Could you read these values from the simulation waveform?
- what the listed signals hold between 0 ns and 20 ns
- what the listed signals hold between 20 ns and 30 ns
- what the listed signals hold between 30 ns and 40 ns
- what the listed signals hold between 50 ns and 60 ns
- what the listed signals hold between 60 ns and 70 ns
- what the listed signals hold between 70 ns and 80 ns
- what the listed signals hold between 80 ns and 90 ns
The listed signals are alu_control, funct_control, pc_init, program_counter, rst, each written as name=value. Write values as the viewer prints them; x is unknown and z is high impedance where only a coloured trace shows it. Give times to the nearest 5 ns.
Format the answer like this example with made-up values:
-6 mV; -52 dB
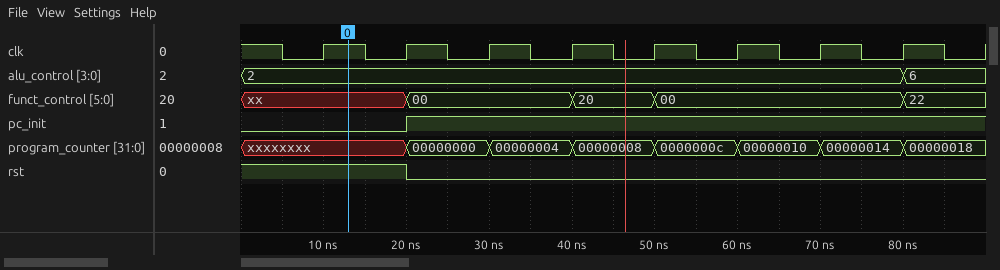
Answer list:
alu_control=2, funct_control=xx, pc_init=0, program_counter=xxxxxxxx, rst=1; alu_control=2, funct_control=00, pc_init=1, program_counter=00000000, rst=0; alu_control=2, funct_control=00, pc_init=1, program_counter=00000004, rst=0; alu_control=2, funct_control=00, pc_init=1, program_counter=0000000c, rst=0; alu_control=2, funct_control=00, pc_init=1, program_counter=00000010, rst=0; alu_control=2, funct_control=00, pc_init=1, program_counter=00000014, rst=0; alu_control=6, funct_control=22, pc_init=1, program_counter=00000018, rst=0
